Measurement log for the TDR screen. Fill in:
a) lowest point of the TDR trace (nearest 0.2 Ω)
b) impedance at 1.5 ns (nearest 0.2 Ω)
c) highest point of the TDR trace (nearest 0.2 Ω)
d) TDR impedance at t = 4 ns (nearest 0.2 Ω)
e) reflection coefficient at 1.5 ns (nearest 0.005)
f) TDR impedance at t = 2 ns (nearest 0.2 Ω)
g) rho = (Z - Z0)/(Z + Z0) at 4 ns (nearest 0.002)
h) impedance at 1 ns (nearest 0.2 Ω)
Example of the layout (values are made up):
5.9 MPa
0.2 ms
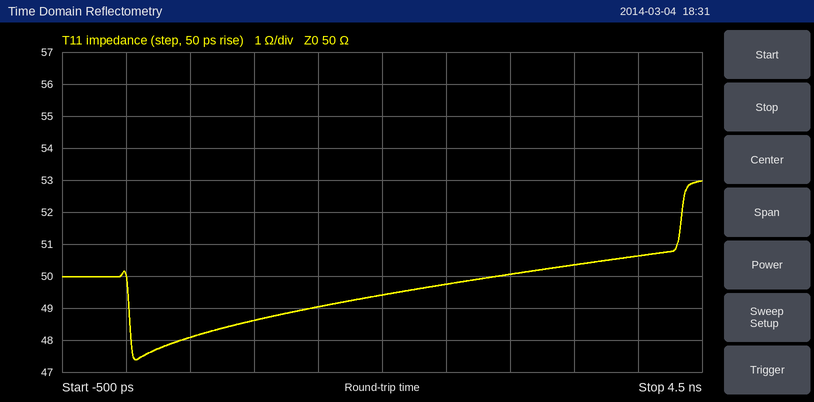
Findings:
47.4 Ω
49.0 Ω
53.0 Ω
50.6 Ω
-0.010
49.4 Ω
+0.006
48.6 Ω
